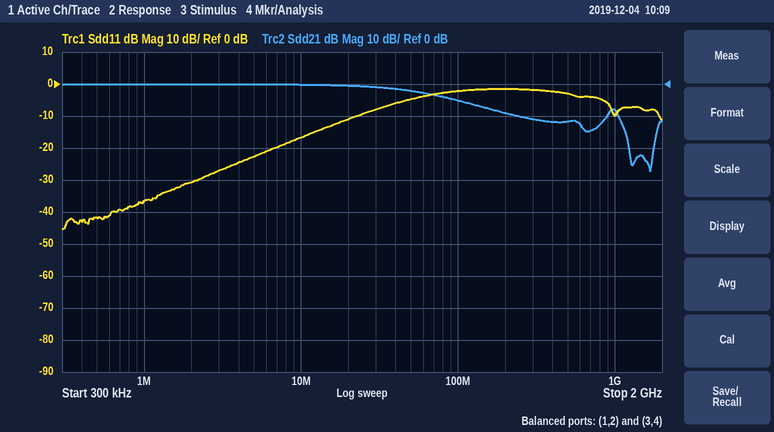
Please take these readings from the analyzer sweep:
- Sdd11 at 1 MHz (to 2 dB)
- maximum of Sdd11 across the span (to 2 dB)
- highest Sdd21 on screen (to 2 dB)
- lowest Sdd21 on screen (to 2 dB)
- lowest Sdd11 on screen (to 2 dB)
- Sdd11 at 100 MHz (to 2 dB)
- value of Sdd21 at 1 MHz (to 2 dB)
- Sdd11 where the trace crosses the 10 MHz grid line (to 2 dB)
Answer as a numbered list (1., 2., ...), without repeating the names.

1. -36 dB
2. -2 dB
3. 0 dB
4. -28 dB
5. -46 dB
6. -2 dB
7. 0 dB
8. -16 dB
